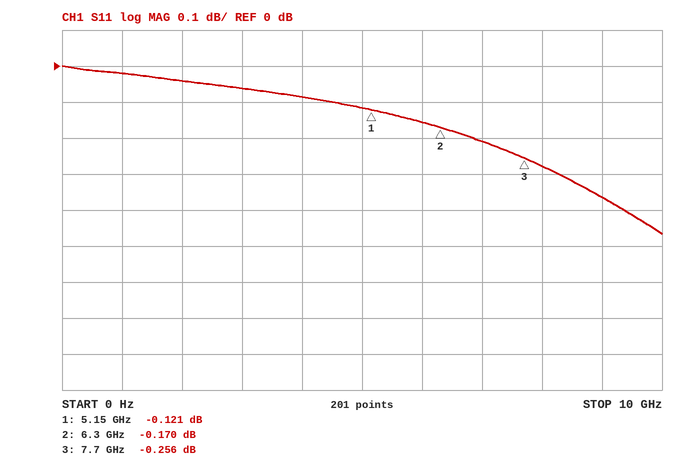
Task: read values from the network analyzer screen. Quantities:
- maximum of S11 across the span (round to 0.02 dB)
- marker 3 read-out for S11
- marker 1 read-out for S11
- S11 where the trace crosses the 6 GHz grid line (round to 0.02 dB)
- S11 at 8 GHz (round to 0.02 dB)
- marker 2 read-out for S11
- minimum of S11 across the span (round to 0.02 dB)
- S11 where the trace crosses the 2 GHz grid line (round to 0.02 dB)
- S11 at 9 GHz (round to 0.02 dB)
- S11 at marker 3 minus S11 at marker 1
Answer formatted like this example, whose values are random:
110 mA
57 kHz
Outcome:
0.00 dB
-0.256 dB
-0.121 dB
-0.16 dB
-0.28 dB
-0.170 dB
-0.46 dB
-0.04 dB
-0.36 dB
-0.135 dB
